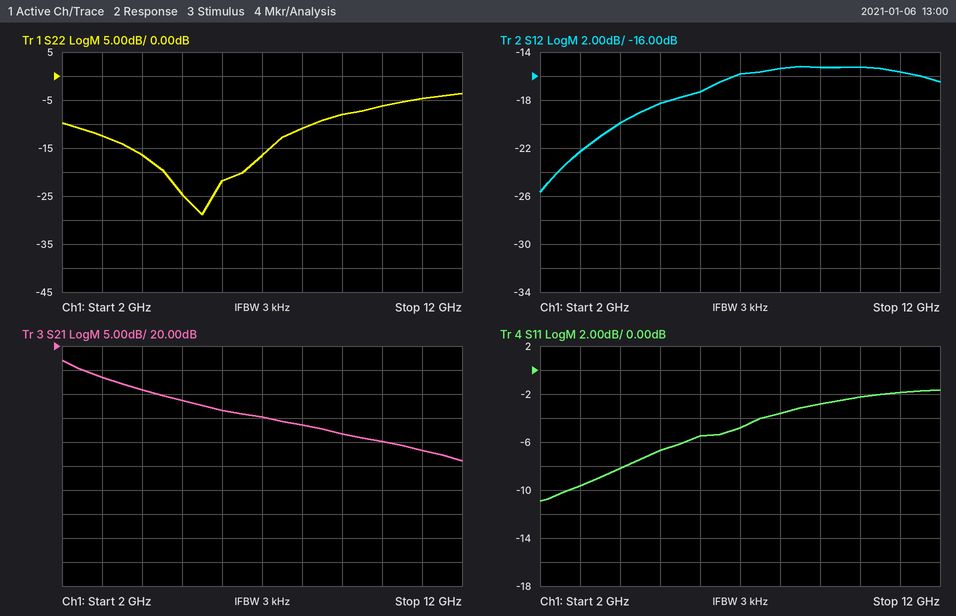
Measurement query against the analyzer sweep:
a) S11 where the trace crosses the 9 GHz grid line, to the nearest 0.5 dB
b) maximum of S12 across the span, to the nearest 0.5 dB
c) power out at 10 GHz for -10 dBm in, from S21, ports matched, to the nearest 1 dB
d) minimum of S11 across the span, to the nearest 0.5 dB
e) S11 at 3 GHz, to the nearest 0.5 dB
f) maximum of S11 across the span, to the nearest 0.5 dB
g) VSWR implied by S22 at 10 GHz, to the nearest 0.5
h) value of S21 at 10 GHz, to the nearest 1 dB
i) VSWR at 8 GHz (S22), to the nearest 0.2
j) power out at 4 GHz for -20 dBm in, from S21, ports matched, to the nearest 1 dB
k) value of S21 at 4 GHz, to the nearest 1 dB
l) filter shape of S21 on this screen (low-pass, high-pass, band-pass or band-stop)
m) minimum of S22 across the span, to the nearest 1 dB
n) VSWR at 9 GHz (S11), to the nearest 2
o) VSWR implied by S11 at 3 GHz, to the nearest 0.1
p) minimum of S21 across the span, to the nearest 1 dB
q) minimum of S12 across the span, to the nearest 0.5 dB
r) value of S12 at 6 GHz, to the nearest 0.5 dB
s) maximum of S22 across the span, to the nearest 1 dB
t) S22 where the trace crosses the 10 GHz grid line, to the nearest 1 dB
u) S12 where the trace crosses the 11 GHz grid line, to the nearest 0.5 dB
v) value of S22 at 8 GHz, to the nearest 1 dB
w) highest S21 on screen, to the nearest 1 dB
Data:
-3.0 dB
-15.0 dB
-10 dBm
-11.0 dB
-9.5 dB
-1.5 dB
3.0
0 dB
1.8
-9 dBm
11 dB
low-pass
-29 dB
6
2.0
-4 dB
-25.5 dB
-17.5 dB
-4 dB
-6 dB
-15.5 dB
-11 dB
17 dB
